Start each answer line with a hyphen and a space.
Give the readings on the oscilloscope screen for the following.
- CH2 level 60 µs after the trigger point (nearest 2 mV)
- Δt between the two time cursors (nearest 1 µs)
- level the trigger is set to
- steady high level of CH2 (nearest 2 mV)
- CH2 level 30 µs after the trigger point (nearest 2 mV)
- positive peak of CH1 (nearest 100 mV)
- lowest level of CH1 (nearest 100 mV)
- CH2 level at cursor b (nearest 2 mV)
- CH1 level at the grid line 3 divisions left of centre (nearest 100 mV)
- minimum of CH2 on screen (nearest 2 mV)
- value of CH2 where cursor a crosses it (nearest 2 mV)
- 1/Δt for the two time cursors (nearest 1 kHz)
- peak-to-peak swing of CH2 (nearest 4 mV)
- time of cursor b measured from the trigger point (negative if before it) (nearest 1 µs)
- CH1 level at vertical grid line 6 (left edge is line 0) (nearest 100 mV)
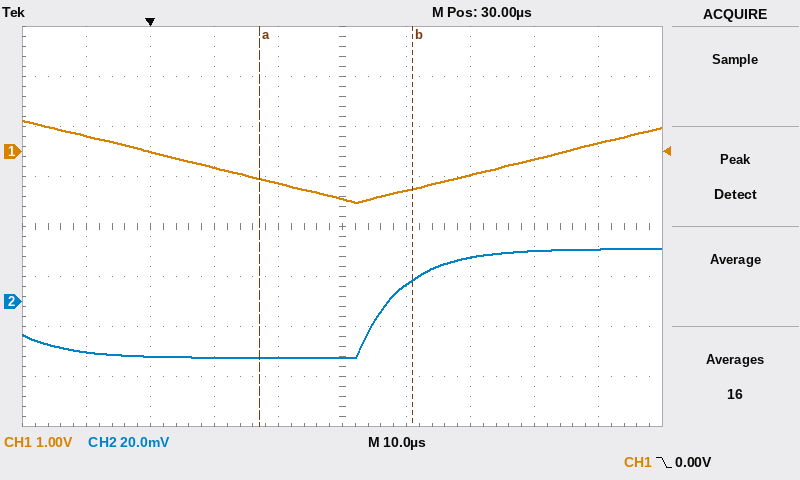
- 20 mV
- 24 µs
- 0.00 V
- 20 mV
- -22 mV
- 600 mV
- -1.0 V
- 8 mV
- 0.0 V
- -22 mV
- -22 mV
- 42 kHz
- 44 mV
- +41 µs
- -800 mV
